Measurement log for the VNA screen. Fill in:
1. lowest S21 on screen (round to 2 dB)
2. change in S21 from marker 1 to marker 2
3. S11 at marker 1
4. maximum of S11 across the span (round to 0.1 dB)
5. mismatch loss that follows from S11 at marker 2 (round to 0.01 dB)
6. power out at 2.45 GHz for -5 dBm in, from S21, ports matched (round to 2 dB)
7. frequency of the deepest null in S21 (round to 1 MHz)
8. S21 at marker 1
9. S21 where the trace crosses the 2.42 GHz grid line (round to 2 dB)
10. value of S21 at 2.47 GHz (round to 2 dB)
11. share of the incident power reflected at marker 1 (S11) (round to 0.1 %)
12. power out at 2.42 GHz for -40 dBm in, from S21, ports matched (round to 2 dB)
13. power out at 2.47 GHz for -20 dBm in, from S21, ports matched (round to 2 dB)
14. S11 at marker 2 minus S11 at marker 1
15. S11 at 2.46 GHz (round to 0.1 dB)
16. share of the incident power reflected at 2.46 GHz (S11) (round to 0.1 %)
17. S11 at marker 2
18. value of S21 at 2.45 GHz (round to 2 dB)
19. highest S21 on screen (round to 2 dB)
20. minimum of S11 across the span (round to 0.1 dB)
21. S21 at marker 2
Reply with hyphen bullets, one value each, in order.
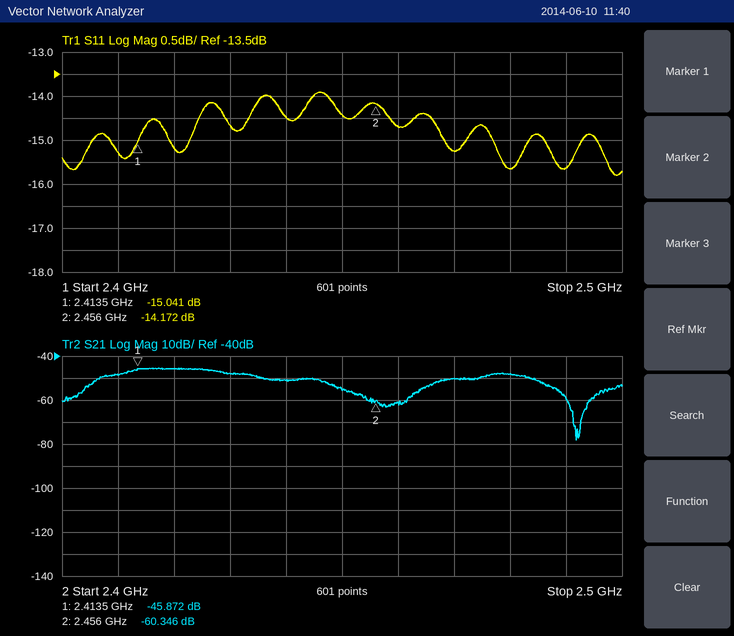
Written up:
- -78 dB
- -14.474 dB
- -15.041 dB
- -13.9 dB
- 0.17 dB
- -60 dBm
- 2.492 GHz
- -45.872 dB
- -46 dB
- -50 dB
- 3.1 %
- -86 dBm
- -70 dBm
- 0.869 dB
- -14.7 dB
- 3.4 %
- -14.172 dB
- -56 dB
- -46 dB
- -15.8 dB
- -60.346 dB
